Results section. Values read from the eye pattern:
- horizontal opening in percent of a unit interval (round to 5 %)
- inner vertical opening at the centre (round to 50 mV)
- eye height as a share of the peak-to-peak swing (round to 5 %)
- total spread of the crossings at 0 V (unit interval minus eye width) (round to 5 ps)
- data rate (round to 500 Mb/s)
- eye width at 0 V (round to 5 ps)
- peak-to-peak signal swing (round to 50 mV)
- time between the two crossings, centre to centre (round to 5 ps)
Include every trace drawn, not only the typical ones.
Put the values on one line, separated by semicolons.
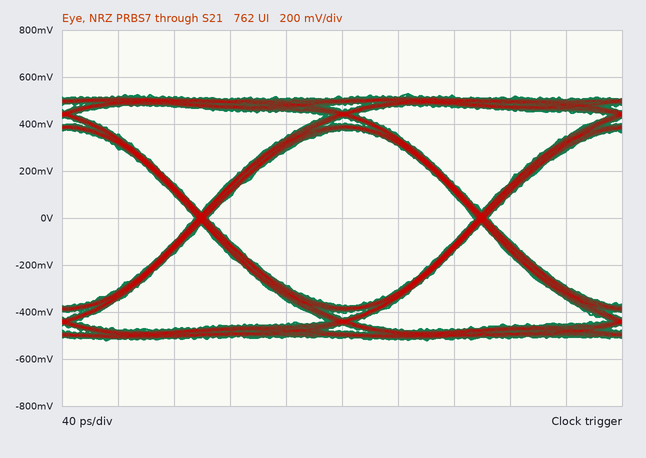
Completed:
95 %; 750 mV; 70 %; 10 ps; 5.0 Gb/s; 190 ps; 1.05 V; 200 ps
